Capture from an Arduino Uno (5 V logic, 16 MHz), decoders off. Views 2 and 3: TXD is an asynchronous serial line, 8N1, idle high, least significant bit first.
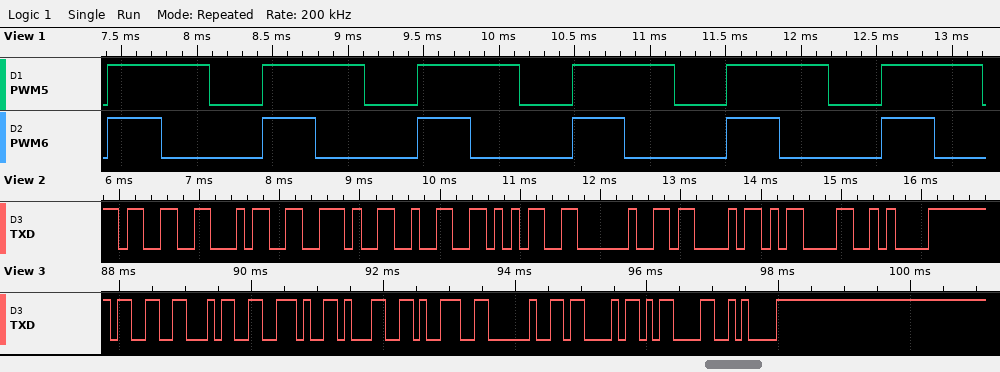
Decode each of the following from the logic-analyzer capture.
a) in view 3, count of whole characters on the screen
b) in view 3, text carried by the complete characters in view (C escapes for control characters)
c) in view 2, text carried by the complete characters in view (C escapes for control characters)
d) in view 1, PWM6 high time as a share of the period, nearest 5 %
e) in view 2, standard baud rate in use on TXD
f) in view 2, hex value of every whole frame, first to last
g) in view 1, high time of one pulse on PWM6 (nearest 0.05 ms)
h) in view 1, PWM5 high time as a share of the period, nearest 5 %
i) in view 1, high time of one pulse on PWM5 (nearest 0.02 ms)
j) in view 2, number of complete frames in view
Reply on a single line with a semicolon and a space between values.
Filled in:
9; "34.19 C\r\n"; "34.25 C\r\n"; 35 %; 9600 baud; 33 34 2E 32 35 20 43 0D 0A; 0.35 ms; 65 %; 0.68 ms; 9
